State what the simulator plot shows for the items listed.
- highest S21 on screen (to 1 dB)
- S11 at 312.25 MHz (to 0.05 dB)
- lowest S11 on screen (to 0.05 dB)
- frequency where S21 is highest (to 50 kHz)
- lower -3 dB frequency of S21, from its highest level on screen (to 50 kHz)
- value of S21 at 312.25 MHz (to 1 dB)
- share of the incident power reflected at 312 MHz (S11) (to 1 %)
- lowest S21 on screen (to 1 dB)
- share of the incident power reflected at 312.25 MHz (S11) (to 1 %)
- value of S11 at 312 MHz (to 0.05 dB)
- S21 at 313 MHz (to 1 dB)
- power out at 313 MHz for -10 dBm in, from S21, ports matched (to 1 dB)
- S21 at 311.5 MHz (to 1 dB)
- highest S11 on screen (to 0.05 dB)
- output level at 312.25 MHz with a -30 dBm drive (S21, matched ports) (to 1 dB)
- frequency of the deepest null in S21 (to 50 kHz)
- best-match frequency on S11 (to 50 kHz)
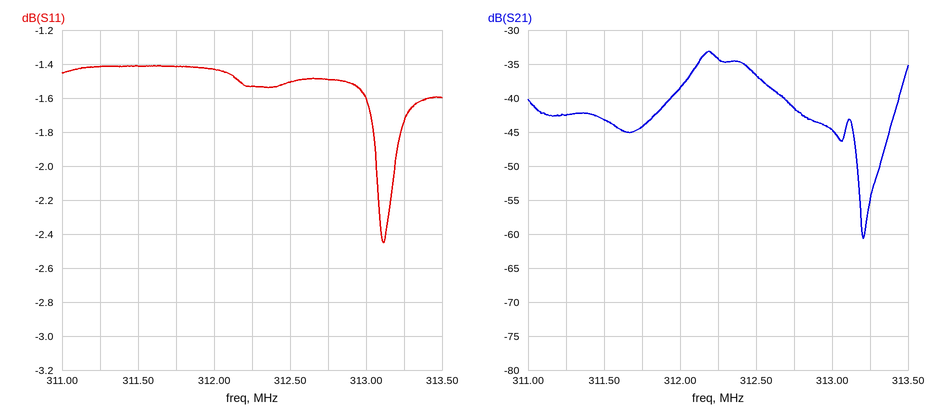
-33 dB
-1.55 dB
-2.45 dB
312.20 MHz
312.10 MHz
-34 dB
72 %
-61 dB
70 %
-1.45 dB
-45 dB
-55 dBm
-43 dB
-1.40 dB
-64 dBm
313.20 MHz
313.10 MHz
